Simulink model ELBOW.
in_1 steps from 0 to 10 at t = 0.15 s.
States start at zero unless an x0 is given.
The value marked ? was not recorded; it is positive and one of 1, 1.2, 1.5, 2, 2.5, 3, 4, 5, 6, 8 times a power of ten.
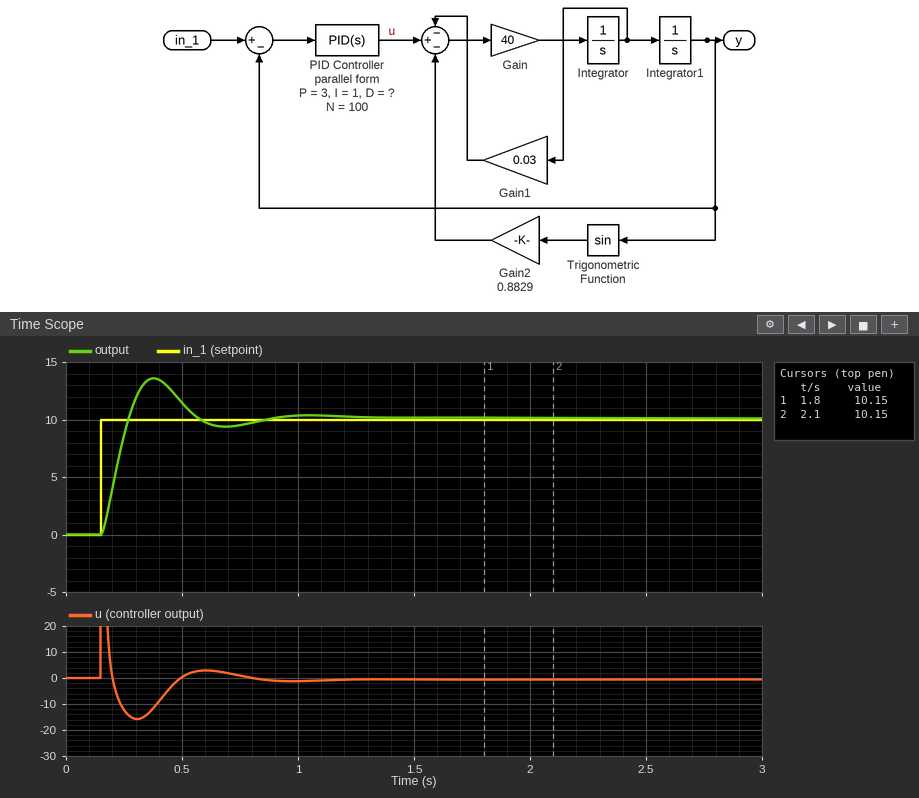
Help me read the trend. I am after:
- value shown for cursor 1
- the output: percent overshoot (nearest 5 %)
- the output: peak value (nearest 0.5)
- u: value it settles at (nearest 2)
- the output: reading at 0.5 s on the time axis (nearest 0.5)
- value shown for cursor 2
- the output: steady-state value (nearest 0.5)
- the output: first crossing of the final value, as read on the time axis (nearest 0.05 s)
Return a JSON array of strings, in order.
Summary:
["10.15", "35 %", "13.5", "0", "11.5", "10.15", "10.0", "0.25 s"]
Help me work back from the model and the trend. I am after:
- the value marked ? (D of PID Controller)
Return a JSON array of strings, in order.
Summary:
["0.2"]
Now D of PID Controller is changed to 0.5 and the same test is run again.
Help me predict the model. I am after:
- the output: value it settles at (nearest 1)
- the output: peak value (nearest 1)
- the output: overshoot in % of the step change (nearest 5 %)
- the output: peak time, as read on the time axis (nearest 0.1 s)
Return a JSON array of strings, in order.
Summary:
["10", "11", "15 %", "0.3 s"]
